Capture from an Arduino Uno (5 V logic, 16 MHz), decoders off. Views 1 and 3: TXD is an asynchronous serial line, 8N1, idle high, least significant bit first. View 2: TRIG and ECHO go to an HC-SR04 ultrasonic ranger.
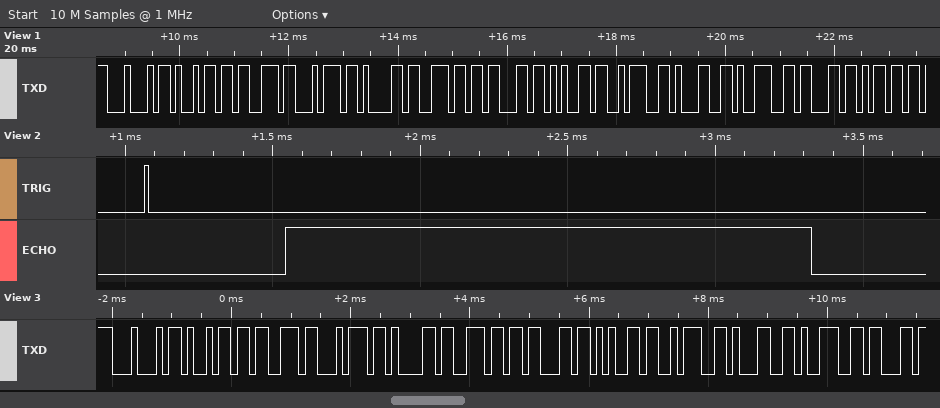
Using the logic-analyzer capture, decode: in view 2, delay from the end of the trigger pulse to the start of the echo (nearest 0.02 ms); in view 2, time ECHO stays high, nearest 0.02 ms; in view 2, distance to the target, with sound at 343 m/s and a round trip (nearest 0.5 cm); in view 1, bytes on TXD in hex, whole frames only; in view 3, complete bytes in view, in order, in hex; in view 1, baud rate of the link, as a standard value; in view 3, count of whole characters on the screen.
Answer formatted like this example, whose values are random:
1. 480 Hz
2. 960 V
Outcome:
1. 0.46 ms
2. 1.78 ms
3. 30.5 cm
4. 44 69 73 74 61 6E 63 65 3A 31 39 63 6D
5. 44 69 73 74 61 6E 63 65 3A 31 39 63
6. 9600 baud
7. 12
